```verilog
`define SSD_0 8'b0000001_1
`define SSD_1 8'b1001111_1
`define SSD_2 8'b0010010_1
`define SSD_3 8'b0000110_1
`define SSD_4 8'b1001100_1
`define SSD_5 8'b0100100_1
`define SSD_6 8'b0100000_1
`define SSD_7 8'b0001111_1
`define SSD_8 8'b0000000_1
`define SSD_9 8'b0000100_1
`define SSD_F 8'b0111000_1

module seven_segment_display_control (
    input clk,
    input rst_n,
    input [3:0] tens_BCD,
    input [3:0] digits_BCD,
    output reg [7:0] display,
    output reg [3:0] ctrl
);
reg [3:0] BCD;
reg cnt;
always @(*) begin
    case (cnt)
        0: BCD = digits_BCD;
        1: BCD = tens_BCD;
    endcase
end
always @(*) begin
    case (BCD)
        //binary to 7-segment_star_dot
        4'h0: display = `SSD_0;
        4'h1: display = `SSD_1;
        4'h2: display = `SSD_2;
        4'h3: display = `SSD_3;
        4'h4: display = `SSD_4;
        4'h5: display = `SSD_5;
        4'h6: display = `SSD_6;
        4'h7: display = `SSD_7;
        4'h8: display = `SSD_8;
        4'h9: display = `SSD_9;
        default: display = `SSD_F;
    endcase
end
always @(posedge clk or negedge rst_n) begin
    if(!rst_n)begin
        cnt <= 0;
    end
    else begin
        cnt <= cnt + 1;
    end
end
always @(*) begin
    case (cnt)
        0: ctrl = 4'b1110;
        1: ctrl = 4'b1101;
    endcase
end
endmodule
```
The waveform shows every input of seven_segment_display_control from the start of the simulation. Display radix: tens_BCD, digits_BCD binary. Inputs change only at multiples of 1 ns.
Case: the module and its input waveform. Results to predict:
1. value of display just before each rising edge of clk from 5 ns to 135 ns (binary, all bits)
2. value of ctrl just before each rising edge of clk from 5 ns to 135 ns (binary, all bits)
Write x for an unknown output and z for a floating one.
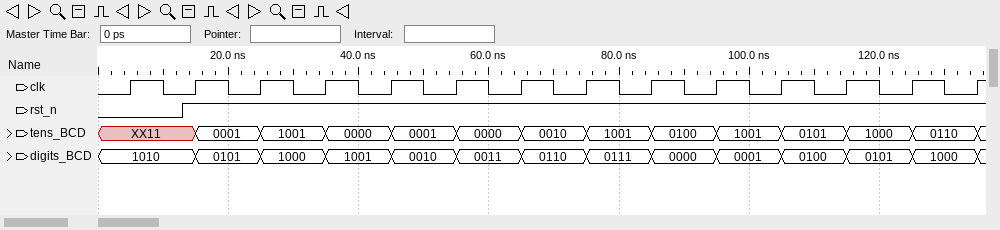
01110001, 01110001, 10011111, 00000001, 00000011, 00100101, 00000011, 01000001, 00001001, 00000011, 00001001, 10011001, 00000001, 00000001
1110, 1110, 1101, 1110, 1101, 1110, 1101, 1110, 1101, 1110, 1101, 1110, 1101, 1110
